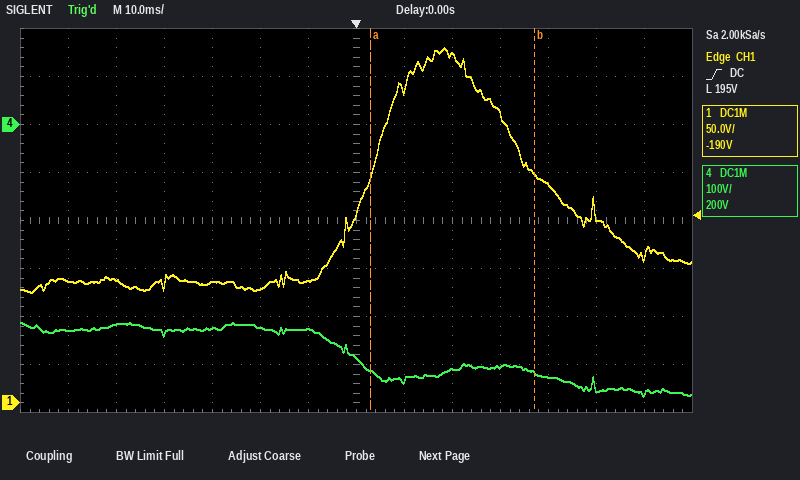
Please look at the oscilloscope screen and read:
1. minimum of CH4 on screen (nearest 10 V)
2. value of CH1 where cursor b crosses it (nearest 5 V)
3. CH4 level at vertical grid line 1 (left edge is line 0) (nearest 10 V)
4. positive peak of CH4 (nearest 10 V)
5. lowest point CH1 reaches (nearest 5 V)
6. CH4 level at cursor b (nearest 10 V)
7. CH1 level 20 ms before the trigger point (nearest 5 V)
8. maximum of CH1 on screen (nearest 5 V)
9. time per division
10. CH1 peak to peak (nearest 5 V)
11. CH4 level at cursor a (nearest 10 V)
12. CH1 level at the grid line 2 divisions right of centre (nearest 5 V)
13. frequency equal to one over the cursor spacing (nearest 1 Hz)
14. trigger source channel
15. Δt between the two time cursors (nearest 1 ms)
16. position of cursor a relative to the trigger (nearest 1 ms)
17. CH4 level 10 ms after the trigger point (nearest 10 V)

-570 V
240 V
-430 V
-410 V
115 V
-520 V
120 V
370 V
10 ms
255 V
-510 V
365 V
29 Hz
CH1
34 ms
+3 ms
-530 V
